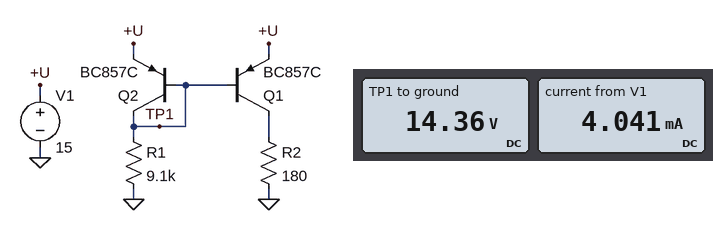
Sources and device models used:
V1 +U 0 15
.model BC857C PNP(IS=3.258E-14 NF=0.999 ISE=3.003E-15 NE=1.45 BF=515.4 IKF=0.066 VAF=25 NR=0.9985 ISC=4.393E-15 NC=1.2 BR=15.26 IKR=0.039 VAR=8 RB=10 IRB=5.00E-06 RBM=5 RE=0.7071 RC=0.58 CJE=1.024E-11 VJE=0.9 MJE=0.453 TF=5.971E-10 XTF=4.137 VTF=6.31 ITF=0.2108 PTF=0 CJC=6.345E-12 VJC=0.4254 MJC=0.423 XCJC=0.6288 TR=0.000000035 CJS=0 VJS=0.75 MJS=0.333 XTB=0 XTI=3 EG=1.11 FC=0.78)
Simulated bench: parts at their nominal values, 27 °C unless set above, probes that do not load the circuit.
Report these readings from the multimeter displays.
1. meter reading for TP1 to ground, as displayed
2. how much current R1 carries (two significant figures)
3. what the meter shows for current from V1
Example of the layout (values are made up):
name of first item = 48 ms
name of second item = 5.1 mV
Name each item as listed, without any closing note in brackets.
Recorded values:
meter reading for TP1 to ground, as displayed = 14.36 V
how much current R1 carries = 1.6 mA
what the meter shows for current from V1 = 4.041 mA
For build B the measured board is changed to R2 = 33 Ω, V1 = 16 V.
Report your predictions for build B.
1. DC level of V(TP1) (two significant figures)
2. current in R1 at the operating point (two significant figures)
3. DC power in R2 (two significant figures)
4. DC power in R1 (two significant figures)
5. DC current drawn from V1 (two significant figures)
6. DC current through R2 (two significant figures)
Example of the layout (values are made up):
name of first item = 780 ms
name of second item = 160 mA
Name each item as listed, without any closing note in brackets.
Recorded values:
DC level of V(TP1) = 15 V
current in R1 at the operating point = 1.7 mA
DC power in R2 = 240 µW
DC power in R1 = 26 mW
DC current drawn from V1 = 4.4 mA
DC current through R2 = 2.7 mA
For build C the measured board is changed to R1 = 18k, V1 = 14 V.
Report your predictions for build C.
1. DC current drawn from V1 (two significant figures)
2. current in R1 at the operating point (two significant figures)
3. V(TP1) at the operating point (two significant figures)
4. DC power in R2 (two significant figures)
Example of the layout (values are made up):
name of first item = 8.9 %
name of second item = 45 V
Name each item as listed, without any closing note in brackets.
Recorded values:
DC current drawn from V1 = 1.9 mA
current in R1 at the operating point = 740 µA
V(TP1) at the operating point = 13 V
DC power in R2 = 240 µW
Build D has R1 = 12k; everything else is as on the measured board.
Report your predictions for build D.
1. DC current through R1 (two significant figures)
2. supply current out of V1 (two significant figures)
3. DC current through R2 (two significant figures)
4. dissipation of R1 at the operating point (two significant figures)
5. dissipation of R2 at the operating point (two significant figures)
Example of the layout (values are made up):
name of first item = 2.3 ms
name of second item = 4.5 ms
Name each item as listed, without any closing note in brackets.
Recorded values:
DC current through R1 = 1.2 mA
supply current out of V1 = 3.1 mA
DC current through R2 = 1.9 mA
dissipation of R1 at the operating point = 17 mW
dissipation of R2 at the operating point = 640 µW
